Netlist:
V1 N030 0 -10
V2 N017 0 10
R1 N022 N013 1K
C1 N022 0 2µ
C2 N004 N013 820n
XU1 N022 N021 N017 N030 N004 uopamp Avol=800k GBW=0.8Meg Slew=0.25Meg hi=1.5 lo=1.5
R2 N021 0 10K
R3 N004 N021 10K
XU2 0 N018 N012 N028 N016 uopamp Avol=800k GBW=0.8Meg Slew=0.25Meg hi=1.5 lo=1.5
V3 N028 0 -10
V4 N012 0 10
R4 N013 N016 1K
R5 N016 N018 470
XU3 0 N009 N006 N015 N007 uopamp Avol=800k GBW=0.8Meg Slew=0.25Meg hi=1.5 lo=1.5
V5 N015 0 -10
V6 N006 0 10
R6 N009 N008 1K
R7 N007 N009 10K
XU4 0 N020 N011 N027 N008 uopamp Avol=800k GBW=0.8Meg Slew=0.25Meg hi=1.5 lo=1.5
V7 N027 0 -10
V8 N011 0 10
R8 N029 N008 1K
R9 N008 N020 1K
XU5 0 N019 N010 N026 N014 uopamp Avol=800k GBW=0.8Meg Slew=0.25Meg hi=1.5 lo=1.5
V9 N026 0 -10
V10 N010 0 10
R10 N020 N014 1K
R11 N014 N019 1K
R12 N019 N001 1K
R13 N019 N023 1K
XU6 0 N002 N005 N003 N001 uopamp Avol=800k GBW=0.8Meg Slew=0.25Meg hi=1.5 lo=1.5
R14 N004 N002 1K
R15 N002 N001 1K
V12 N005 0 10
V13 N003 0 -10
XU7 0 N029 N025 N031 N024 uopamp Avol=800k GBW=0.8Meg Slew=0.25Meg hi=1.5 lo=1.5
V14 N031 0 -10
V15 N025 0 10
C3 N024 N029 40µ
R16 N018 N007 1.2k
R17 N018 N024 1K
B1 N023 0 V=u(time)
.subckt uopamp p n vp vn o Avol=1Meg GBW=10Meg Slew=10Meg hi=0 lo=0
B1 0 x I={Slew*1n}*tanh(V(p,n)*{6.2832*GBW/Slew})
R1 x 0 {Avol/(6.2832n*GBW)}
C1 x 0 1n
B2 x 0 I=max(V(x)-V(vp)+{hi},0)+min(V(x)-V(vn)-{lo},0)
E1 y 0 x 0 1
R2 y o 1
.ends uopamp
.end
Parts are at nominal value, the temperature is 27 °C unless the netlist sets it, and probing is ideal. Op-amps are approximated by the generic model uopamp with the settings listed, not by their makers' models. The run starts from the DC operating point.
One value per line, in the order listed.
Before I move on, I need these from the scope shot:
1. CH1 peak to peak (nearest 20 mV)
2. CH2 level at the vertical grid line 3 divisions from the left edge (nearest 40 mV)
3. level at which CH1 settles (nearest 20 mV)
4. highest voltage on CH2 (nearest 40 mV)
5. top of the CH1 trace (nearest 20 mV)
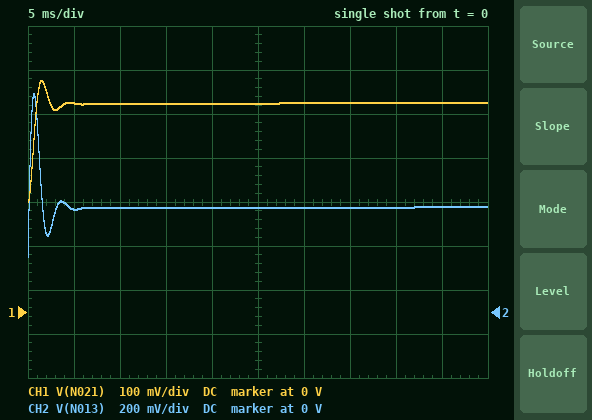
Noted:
280 mV
480 mV
480 mV
1.00 V
520 mV
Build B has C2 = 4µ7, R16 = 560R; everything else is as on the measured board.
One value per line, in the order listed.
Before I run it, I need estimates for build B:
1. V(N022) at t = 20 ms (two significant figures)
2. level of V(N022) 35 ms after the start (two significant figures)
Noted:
790 mV
-710 mV
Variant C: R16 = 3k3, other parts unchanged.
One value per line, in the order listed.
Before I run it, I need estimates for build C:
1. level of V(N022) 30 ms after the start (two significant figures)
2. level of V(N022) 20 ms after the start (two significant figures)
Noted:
450 mV
440 mV
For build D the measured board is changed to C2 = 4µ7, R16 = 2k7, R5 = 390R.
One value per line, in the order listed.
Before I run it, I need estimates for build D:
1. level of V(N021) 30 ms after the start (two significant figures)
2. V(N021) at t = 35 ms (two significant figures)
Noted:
-210 mV
1.2 V
